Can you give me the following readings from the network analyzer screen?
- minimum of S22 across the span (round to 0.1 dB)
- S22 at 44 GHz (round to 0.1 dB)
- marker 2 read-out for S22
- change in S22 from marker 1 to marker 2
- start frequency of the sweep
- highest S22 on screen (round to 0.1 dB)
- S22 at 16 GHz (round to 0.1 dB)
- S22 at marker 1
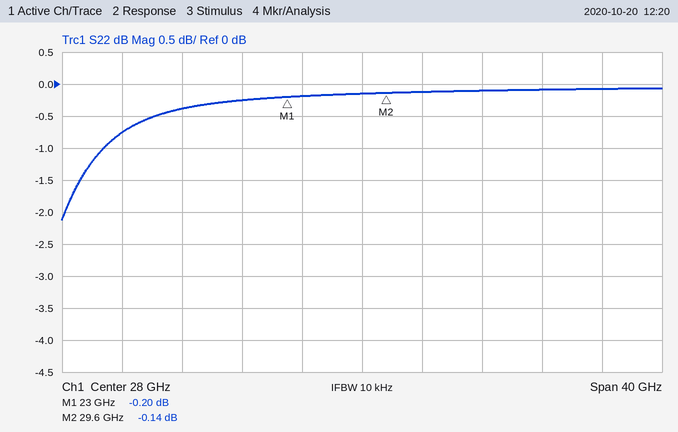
-2.1 dB
-0.1 dB
-0.14 dB
0.06 dB
8 GHz
-0.1 dB
-0.4 dB
-0.20 dB
